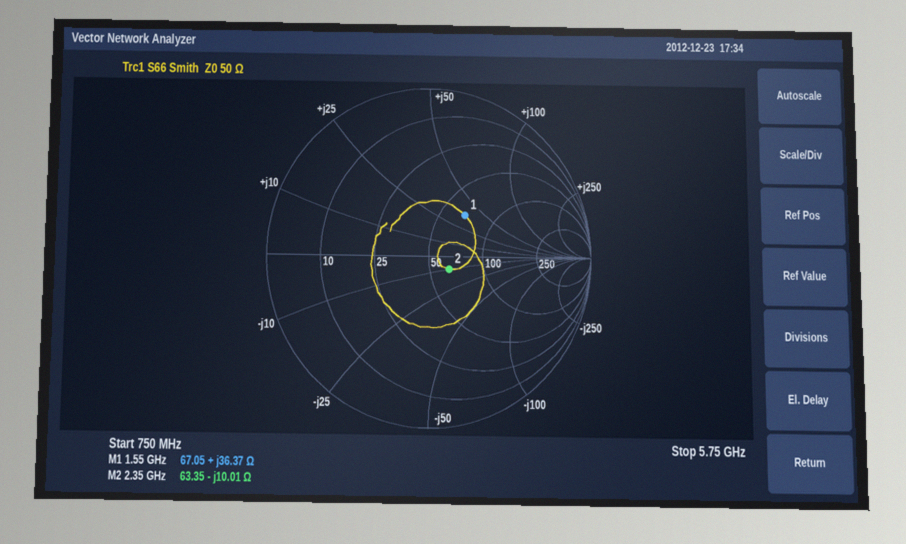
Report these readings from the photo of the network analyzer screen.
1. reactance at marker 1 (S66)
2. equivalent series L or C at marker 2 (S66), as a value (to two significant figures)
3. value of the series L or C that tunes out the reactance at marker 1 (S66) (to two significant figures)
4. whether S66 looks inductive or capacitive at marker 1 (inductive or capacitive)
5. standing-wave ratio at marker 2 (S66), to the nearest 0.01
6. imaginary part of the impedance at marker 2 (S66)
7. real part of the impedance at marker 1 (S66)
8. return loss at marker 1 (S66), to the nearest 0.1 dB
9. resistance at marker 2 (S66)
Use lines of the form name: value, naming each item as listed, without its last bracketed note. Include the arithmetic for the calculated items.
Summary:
reactance at marker 1: +36.37 Ω
equivalent series L or C at marker 2 (S66), as a value: C = 1/(2π × 2.35 GHz × 10.01 Ω) ≈ 6.8 pF
value of the series L or C that tunes out the reactance at marker 1 (S66): C = 1/(2π × 1.55 GHz × 36.37 Ω) ≈ 2.8 pF
whether S66 looks inductive or capacitive at marker 1: inductive
standing-wave ratio at marker 2 (S66), to the nearest 0.01: 1.34
imaginary part of the impedance at marker 2: -10.01 Ω
real part of the impedance at marker 1: 67.05 Ω
return loss at marker 1 (S66), to the nearest 0.1 dB: 9.7 dB
resistance at marker 2: 63.35 Ω
